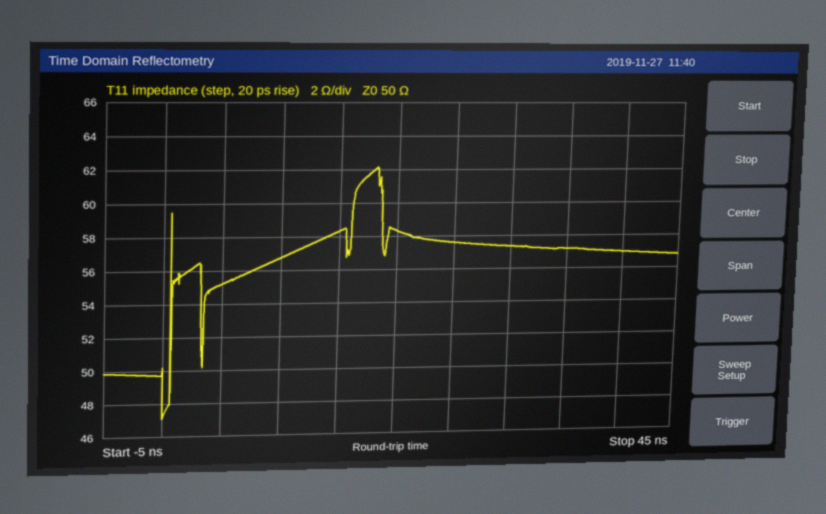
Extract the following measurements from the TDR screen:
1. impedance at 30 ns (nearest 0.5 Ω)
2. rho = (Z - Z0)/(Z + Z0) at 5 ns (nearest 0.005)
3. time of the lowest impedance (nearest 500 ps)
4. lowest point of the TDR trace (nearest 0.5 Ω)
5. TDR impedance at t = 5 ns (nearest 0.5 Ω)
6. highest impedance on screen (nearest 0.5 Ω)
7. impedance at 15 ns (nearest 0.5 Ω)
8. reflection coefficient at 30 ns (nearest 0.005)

57.5 Ω
+0.050
0.0 ns
47.0 Ω
55.0 Ω
62.0 Ω
58.5 Ω
+0.070
